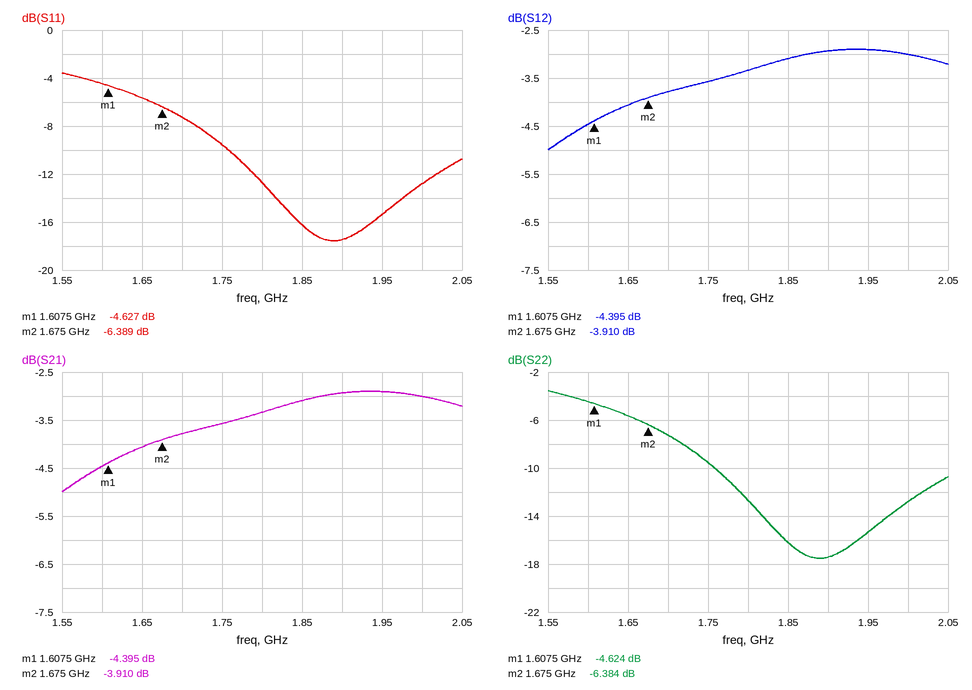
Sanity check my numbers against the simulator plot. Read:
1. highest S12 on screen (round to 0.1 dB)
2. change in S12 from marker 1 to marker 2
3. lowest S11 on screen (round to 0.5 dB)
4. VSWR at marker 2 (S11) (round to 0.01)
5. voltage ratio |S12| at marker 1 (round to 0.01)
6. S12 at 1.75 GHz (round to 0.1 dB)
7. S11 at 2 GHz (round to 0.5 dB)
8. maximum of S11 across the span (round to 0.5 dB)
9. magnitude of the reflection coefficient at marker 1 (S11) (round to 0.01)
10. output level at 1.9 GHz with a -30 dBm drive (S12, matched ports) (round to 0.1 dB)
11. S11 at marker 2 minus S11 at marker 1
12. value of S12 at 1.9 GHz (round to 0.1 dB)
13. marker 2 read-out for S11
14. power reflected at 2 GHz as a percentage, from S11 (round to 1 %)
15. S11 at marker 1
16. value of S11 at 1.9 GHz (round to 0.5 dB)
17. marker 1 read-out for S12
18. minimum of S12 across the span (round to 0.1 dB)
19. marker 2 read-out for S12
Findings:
-2.9 dB
0.485 dB
-17.5 dB
2.84
0.60
-3.6 dB
-13.0 dB
-3.5 dB
0.59
-32.9 dBm
-1.762 dB
-2.9 dB
-6.389 dB
5 %
-4.627 dB
-17.5 dB
-4.395 dB
-5.0 dB
-3.910 dB
